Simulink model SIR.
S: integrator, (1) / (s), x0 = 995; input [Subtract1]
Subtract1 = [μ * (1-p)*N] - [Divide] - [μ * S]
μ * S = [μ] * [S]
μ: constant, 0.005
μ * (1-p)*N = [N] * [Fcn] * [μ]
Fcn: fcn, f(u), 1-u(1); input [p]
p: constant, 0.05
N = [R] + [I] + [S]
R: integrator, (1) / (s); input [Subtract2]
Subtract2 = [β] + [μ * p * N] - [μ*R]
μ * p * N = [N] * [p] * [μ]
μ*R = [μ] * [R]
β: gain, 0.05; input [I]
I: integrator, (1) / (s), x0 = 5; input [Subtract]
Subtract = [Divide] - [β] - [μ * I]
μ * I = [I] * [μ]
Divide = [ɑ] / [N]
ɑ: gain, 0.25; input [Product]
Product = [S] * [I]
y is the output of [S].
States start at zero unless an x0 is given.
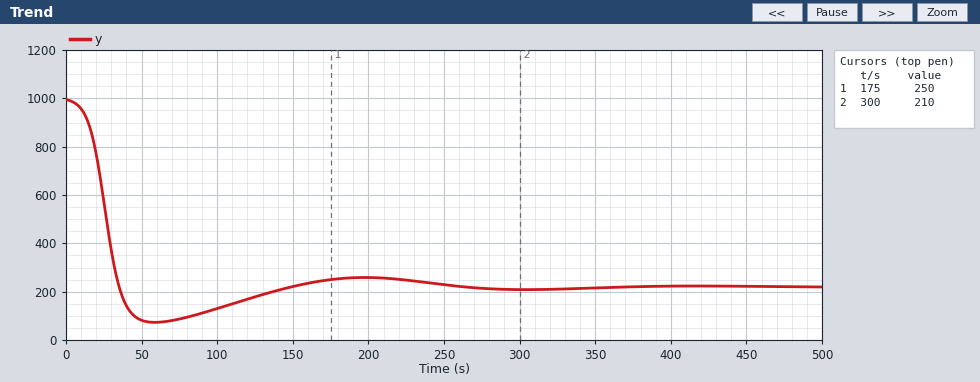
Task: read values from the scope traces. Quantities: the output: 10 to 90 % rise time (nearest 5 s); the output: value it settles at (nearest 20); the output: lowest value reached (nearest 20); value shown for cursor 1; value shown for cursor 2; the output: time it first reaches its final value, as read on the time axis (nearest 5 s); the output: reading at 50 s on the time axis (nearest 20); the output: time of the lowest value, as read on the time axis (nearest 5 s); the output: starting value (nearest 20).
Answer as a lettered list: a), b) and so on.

a) 20 s
b) 220
c) 80
d) 250
e) 210
f) 35 s
g) 80
h) 60 s
i) 1000
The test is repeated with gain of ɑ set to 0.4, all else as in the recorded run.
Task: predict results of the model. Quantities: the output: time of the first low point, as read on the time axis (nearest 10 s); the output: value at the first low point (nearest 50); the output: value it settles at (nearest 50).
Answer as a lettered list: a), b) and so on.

a) 40 s
b) 50
c) 150
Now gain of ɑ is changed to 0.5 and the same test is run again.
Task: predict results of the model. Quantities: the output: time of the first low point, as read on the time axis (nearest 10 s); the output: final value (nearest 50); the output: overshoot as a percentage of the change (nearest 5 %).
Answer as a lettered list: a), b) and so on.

a) 30 s
b) 100
c) 10 %
